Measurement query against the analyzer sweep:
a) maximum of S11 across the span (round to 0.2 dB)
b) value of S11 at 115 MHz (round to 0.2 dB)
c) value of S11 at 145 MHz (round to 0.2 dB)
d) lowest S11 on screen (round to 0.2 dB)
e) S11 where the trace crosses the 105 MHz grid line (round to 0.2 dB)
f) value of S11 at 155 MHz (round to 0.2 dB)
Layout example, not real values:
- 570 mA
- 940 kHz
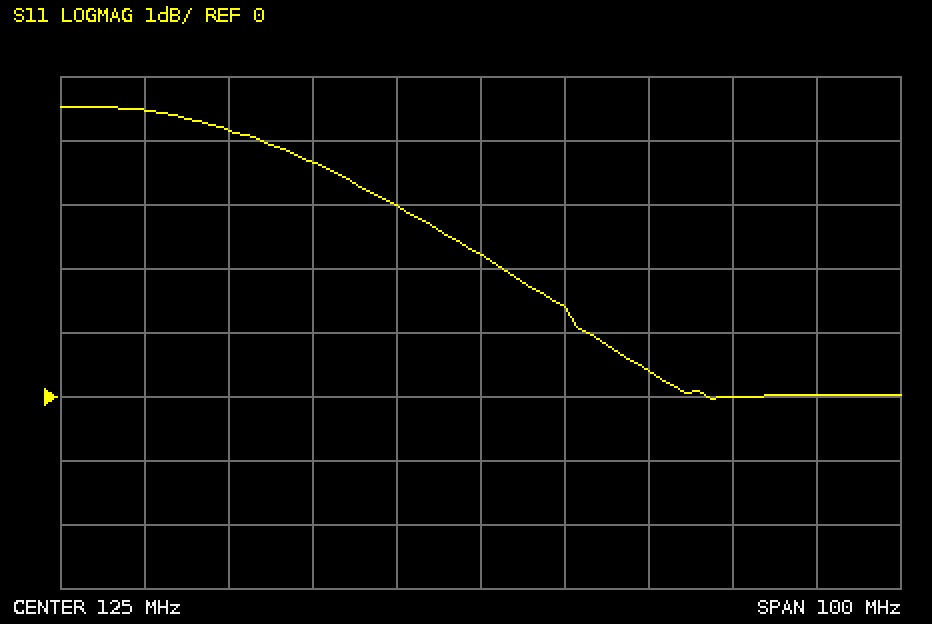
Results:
- 4.6 dB
- 3.0 dB
- 0.4 dB
- 0.0 dB
- 3.6 dB
- 0.0 dB
